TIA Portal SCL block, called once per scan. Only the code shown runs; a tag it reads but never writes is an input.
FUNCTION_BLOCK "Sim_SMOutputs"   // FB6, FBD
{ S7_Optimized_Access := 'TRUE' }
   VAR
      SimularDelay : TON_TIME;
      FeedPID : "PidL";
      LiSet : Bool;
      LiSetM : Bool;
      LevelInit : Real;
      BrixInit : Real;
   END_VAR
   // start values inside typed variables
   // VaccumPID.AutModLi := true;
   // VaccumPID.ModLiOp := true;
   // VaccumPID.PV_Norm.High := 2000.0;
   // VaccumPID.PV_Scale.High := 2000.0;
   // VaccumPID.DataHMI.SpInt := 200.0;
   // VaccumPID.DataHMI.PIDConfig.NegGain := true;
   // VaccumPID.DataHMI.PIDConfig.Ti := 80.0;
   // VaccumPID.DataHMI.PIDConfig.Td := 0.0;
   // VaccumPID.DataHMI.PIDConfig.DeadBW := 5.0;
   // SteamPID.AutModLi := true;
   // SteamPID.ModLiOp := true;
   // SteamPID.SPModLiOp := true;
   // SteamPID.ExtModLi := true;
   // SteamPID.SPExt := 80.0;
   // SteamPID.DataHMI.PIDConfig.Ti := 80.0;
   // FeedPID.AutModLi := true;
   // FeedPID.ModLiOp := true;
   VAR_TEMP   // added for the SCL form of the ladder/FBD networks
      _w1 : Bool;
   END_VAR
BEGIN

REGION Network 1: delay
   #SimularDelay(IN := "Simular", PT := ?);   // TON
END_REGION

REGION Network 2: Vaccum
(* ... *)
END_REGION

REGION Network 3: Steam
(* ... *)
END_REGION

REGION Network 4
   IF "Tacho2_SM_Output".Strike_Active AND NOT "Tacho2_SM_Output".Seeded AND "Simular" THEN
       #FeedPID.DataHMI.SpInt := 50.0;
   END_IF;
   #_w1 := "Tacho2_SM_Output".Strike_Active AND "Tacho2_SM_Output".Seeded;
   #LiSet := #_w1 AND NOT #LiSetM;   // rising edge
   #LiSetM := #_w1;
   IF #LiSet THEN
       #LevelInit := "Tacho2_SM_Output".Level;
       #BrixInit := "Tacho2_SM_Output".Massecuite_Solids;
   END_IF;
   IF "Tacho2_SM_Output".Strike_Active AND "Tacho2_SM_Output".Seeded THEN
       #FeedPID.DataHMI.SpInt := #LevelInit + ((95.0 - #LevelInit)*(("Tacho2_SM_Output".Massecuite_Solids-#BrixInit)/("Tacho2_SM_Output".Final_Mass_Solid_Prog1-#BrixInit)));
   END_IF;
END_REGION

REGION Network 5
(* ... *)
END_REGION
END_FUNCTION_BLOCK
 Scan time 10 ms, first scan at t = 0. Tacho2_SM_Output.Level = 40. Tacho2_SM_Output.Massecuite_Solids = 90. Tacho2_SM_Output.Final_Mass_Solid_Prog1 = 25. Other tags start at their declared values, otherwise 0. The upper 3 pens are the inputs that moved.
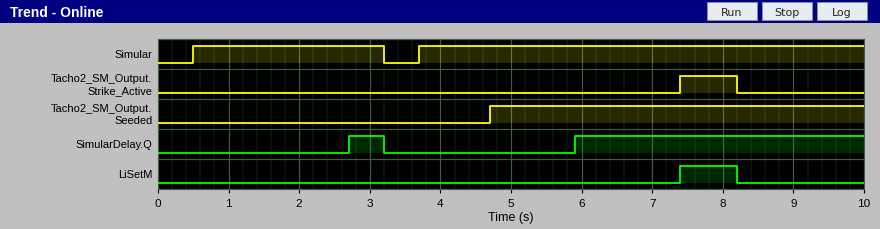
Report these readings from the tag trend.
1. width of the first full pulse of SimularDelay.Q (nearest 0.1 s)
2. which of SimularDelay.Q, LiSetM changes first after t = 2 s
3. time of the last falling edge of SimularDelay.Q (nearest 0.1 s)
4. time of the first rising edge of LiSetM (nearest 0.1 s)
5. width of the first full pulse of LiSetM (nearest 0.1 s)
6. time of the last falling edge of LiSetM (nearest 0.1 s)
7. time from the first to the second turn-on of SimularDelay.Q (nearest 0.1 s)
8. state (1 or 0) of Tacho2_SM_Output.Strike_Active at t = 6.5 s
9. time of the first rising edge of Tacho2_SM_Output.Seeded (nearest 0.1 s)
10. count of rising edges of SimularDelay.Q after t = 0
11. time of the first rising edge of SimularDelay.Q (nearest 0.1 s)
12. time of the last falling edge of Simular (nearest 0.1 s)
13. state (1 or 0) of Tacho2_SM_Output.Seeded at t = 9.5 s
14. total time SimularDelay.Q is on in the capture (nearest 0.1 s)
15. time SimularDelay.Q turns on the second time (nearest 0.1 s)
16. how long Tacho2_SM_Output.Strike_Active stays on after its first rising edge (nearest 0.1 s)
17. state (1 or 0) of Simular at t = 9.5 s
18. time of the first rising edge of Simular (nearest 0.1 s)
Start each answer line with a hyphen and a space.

- 0.5 s
- SimularDelay.Q
- 3.2 s
- 7.4 s
- 0.8 s
- 8.2 s
- 3.2 s
- 0
- 4.7 s
- 2
- 2.7 s
- 3.2 s
- 1
- 4.6 s
- 5.9 s
- 0.8 s
- 1
- 0.5 s
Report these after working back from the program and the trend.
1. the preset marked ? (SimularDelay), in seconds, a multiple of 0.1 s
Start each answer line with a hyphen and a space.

- 2.2 s
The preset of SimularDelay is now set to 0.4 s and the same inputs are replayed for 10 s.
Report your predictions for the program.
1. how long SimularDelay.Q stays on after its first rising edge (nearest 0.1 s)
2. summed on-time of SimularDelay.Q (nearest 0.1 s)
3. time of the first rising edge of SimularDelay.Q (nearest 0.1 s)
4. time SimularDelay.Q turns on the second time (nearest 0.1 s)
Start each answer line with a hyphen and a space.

- 2.3 s
- 8.2 s
- 0.9 s
- 4.1 s
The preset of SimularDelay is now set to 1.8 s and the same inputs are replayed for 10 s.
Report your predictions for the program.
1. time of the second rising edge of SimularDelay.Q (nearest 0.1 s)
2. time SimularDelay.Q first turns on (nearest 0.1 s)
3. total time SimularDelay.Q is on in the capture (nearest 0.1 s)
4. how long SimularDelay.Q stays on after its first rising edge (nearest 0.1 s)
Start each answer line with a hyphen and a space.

- 5.5 s
- 2.3 s
- 5.4 s
- 0.9 s
